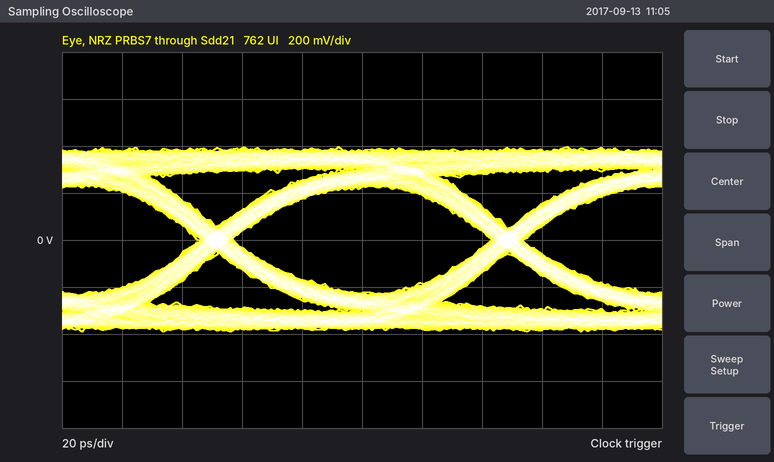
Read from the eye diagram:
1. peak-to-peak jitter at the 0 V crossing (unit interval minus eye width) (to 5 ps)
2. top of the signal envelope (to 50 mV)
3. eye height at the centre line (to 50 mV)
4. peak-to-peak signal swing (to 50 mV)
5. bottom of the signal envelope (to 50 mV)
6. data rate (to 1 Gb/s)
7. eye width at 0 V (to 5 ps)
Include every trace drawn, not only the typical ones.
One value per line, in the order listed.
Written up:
10 ps
400 mV
450 mV
800 mV
-400 mV
10 Gb/s
85 ps
